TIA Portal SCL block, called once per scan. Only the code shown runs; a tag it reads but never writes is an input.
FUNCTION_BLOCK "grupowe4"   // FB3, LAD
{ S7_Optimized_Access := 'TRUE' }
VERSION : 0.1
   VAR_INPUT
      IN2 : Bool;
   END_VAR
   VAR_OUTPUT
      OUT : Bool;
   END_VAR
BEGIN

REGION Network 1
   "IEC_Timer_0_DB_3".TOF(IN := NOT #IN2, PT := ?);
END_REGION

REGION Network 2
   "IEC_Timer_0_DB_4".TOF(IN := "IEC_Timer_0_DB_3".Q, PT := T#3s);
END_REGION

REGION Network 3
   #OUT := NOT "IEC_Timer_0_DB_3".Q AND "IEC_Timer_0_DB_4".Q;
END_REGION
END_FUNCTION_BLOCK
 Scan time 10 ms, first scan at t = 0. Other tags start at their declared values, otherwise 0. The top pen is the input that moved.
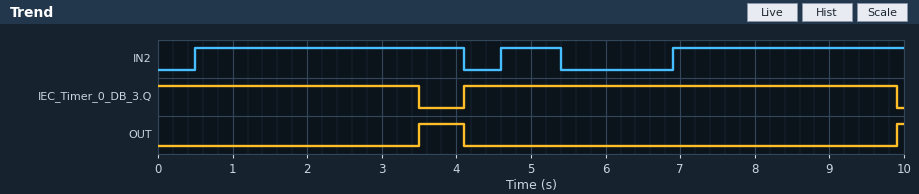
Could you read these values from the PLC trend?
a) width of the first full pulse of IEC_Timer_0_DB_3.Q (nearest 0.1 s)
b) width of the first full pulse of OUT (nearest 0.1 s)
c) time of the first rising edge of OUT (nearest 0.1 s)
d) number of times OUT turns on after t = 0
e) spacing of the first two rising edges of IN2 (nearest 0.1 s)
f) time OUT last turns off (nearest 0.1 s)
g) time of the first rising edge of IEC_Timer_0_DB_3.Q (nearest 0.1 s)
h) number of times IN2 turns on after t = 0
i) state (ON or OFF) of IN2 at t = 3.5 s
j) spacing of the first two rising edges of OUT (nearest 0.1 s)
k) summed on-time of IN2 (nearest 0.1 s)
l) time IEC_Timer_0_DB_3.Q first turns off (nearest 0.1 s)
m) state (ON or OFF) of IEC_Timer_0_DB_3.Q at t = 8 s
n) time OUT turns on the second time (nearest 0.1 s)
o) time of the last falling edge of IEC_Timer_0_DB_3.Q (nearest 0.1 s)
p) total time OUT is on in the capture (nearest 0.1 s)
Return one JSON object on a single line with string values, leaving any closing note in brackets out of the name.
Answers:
{"width of the first full pulse of IEC_Timer_0_DB_3.Q": "5.8 s", "width of the first full pulse of OUT": "0.6 s", "time of the first rising edge of OUT": "3.5 s", "number of times OUT turns on after t = 0": "2", "spacing of the first two rising edges of IN2": "4.1 s", "time OUT last turns off": "4.1 s", "time of the first rising edge of IEC_Timer_0_DB_3.Q": "4.1 s", "number of times IN2 turns on after t = 0": "3", "state (ON or OFF) of IN2 at t = 3.5 s": "ON", "spacing of the first two rising edges of OUT": "6.4 s", "summed on-time of IN2": "7.5 s", "time IEC_Timer_0_DB_3.Q first turns off": "3.5 s", "state (ON or OFF) of IEC_Timer_0_DB_3.Q at t = 8 s": "ON", "time OUT turns on the second time": "9.9 s", "time of the last falling edge of IEC_Timer_0_DB_3.Q": "9.9 s", "total time OUT is on in the capture": "0.7 s"}
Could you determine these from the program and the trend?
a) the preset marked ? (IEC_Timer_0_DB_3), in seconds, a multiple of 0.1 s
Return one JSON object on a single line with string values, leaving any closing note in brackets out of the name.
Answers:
{"the preset marked ? (IEC_Timer_0_DB_3), in seconds, a multiple of 0.1 s": "3.0 s"}
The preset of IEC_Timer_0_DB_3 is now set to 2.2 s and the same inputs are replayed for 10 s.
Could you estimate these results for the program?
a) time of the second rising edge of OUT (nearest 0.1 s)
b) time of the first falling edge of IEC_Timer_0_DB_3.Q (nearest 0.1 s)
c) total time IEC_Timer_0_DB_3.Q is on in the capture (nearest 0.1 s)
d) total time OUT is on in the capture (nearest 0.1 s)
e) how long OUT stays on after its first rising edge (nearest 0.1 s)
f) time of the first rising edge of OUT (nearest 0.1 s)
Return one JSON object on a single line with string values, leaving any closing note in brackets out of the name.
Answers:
{"time of the second rising edge of OUT": "9.1 s", "time of the first falling edge of IEC_Timer_0_DB_3.Q": "2.7 s", "total time IEC_Timer_0_DB_3.Q is on in the capture": "7.7 s", "total time OUT is on in the capture": "2.3 s", "how long OUT stays on after its first rising edge": "1.4 s", "time of the first rising edge of OUT": "2.7 s"}
